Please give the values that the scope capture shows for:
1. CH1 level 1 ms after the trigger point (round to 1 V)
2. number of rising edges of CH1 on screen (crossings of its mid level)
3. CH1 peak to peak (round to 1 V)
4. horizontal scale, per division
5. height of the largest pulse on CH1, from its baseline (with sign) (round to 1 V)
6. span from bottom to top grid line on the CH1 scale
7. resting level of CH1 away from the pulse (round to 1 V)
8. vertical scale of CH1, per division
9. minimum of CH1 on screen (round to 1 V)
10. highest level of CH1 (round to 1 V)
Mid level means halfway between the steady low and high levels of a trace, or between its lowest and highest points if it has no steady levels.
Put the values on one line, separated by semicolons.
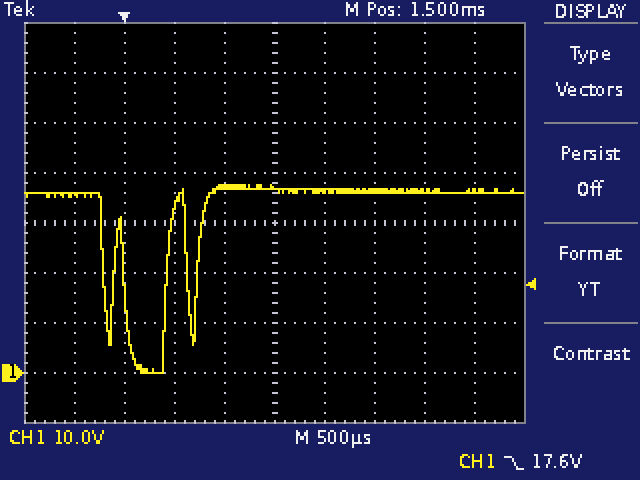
37 V; 3; 38 V; 500 µs; -36 V; 80 V; 36 V; 10 V; 0 V; 38 V
